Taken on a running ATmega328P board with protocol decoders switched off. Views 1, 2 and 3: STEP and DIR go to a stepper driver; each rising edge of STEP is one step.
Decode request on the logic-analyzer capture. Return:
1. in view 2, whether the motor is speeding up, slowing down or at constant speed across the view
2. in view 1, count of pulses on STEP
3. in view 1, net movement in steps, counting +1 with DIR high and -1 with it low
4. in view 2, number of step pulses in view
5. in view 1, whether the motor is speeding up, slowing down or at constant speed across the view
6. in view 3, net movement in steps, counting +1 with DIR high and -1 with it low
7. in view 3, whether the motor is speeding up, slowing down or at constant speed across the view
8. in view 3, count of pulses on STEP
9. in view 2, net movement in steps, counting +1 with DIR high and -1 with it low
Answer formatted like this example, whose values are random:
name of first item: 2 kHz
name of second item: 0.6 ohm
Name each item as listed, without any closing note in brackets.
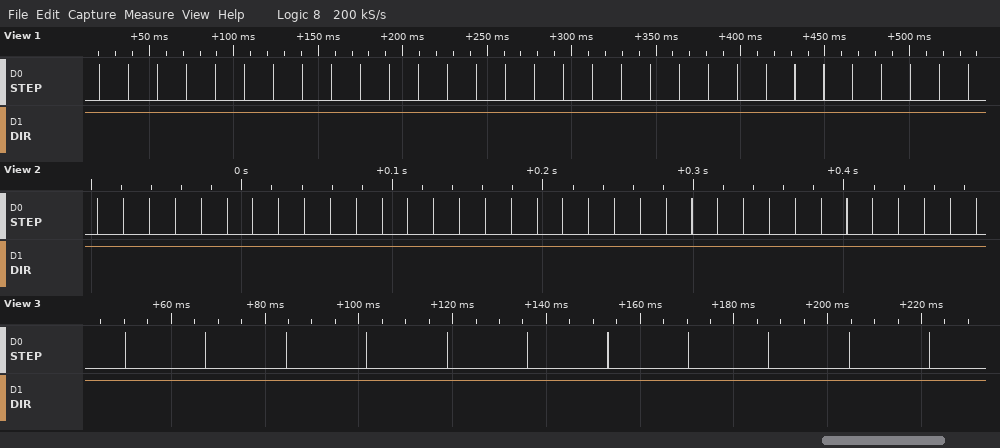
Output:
in view 2, whether the motor is speeding up, slowing down or at constant speed across the view: constant speed
in view 1, count of pulses on STEP: 31
in view 1, net movement in steps, counting +1 with DIR high and -1 with it low: +31
in view 2, number of step pulses in view: 35
in view 1, whether the motor is speeding up, slowing down or at constant speed across the view: constant speed
in view 3, net movement in steps, counting +1 with DIR high and -1 with it low: +11
in view 3, whether the motor is speeding up, slowing down or at constant speed across the view: constant speed
in view 3, count of pulses on STEP: 11
in view 2, net movement in steps, counting +1 with DIR high and -1 with it low: +35
